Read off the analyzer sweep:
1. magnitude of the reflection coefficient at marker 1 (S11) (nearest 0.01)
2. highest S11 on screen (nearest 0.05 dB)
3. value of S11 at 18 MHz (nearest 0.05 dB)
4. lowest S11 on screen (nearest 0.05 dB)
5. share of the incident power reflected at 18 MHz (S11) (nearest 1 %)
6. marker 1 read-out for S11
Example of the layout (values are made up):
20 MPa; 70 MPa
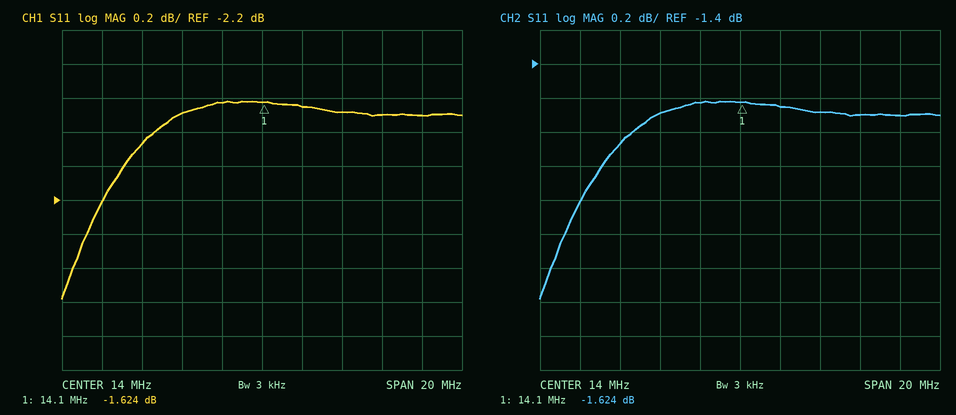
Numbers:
0.83; -1.60 dB; -1.70 dB; -2.80 dB; 68 %; -1.624 dB
